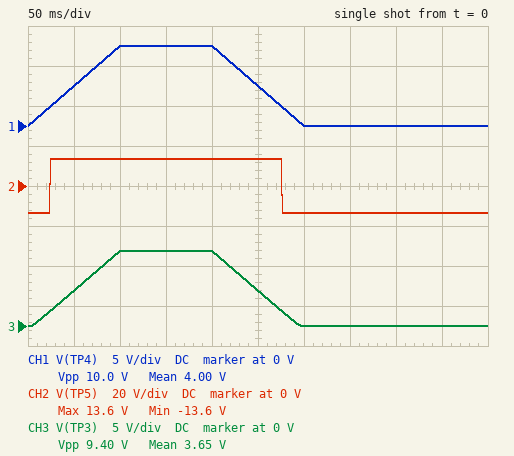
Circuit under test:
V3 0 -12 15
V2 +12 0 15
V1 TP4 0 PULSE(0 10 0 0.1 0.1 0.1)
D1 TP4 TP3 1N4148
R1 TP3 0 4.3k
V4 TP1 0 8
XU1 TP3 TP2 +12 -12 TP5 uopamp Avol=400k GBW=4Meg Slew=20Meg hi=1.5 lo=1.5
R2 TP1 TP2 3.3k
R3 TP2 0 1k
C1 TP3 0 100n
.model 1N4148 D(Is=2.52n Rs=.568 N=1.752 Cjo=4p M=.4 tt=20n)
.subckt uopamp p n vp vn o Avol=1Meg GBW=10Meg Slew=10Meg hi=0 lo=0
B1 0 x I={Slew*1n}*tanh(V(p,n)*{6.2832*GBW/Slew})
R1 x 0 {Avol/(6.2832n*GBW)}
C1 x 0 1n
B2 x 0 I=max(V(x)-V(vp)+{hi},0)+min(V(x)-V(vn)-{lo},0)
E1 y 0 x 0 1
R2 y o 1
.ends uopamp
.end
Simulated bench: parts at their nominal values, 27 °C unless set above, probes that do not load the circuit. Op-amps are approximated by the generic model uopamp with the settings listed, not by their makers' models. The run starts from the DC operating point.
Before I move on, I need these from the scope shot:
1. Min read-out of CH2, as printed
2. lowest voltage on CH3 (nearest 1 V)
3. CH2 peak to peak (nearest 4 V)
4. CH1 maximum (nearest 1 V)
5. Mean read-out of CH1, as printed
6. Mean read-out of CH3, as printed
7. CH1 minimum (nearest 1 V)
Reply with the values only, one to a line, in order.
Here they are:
-13.6 V
0 V
28 V
10 V
4.00 V
3.65 V
0 V
